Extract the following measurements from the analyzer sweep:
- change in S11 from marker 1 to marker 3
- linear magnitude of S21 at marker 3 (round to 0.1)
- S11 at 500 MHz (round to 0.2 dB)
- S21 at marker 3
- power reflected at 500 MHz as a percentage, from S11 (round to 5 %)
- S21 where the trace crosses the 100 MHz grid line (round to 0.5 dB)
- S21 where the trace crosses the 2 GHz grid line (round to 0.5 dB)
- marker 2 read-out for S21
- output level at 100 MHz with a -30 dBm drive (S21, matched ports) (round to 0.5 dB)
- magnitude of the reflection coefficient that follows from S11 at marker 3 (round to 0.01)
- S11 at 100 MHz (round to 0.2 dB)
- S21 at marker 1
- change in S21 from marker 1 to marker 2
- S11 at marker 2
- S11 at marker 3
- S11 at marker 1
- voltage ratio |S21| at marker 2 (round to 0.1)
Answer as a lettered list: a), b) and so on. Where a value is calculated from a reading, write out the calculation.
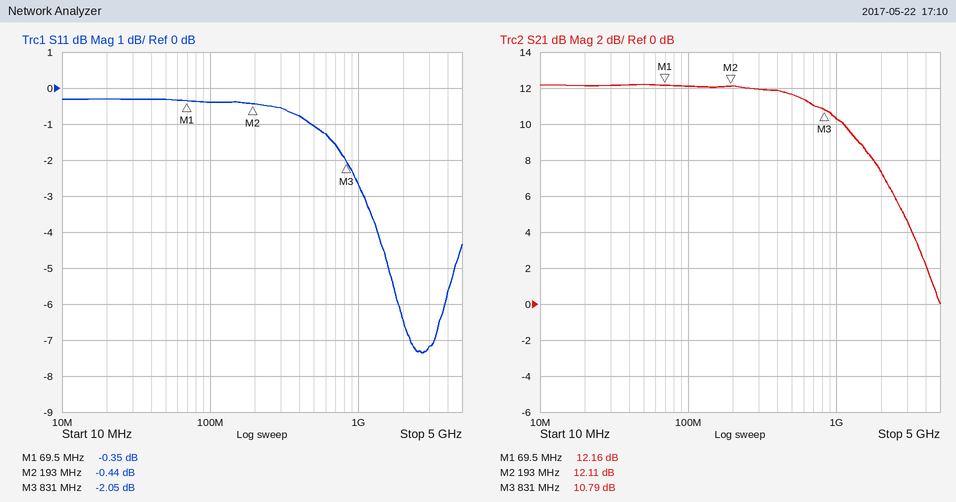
a) -2.05 − (-0.35) = -1.70 dB
b) 10^(10.79/20) ≈ 3.5
c) -1.0 dB
d) 10.79 dB
e) 10^(-1/10) ≈ 79.4 %, so 80 % to the nearest 5 %
f) 12.0 dB
g) 7.5 dB
h) 12.11 dB
i) -30 dBm + (12.0 dB) = -18.0 dBm
j) 10^(-2.05/20) ≈ 0.79
k) -0.4 dB
l) 12.16 dB
m) 12.11 − (12.16) = -0.05 dB
n) -0.44 dB
o) -2.05 dB
p) -0.35 dB
q) 10^(12.11/20) ≈ 4.0
